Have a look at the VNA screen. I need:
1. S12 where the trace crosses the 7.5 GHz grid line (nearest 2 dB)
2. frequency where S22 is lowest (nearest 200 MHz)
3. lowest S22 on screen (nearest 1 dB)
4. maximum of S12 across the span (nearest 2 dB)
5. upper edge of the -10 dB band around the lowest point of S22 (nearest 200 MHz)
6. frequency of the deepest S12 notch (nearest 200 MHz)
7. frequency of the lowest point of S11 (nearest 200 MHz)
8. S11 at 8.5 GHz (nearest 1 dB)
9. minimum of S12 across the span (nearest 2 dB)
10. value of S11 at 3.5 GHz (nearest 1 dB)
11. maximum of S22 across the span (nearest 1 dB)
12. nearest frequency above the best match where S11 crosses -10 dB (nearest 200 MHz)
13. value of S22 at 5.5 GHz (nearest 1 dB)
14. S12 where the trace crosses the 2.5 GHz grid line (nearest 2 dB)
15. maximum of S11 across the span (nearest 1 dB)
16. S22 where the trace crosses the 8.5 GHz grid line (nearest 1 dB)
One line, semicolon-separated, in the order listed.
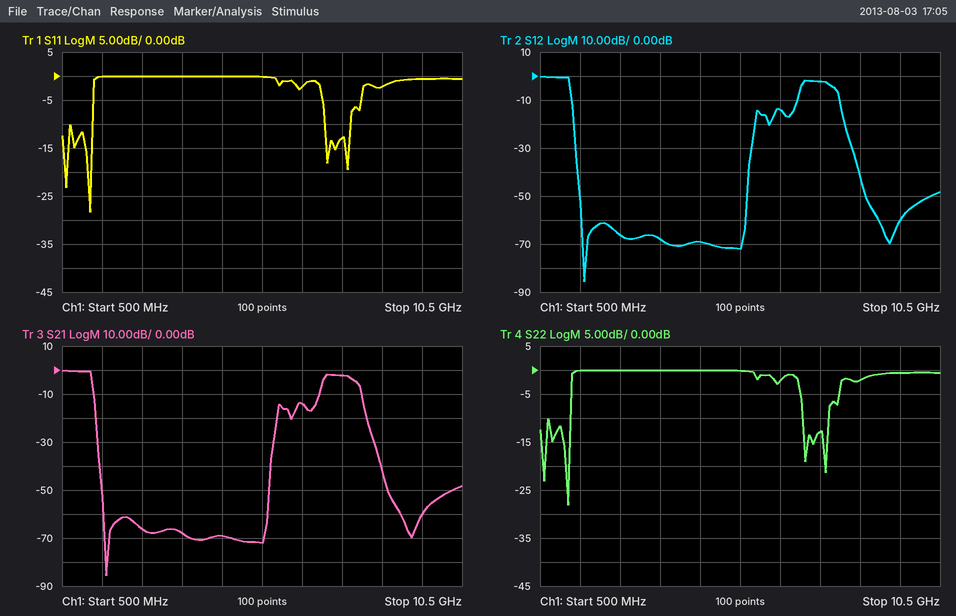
-2 dB; 1.2 GHz; -28 dB; 0 dB; 1.2 GHz; 1.6 GHz; 1.2 GHz; -2 dB; -86 dB; 0 dB; 0 dB; 1.2 GHz; 0 dB; -66 dB; 0 dB; -2 dB
